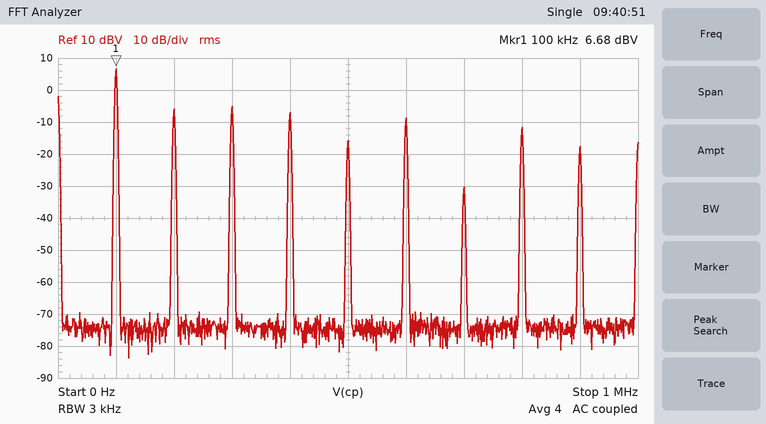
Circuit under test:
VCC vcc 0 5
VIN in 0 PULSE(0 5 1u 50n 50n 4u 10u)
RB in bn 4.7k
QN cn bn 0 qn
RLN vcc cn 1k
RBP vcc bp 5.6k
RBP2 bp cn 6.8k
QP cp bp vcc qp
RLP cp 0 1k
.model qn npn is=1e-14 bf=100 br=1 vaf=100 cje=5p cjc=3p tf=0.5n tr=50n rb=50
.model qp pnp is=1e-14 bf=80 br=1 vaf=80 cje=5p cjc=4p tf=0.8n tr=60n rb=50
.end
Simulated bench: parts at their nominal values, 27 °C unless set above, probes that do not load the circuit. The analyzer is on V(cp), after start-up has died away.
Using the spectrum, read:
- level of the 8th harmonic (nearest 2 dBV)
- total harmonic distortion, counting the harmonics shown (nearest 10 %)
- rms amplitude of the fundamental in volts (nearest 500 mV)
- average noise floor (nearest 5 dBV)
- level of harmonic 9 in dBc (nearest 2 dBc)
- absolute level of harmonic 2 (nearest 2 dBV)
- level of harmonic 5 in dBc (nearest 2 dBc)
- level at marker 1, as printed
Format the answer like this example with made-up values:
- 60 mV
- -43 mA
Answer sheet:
- -12 dBV
- 50 %
- 2.0 V
- -75 dBV
- -24 dBc
- -6 dBV
- -22 dBc
- 6.68 dBV
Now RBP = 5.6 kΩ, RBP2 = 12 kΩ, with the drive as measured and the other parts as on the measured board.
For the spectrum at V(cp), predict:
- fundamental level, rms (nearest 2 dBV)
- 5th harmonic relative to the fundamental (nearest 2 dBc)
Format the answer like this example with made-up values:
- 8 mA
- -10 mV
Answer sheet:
- 6 dBV
- -24 dBc
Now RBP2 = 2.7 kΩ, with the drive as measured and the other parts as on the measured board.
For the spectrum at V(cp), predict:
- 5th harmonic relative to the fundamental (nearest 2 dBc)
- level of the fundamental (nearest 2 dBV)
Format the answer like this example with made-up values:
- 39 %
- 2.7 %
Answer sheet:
- -22 dBc
- 6 dBV
